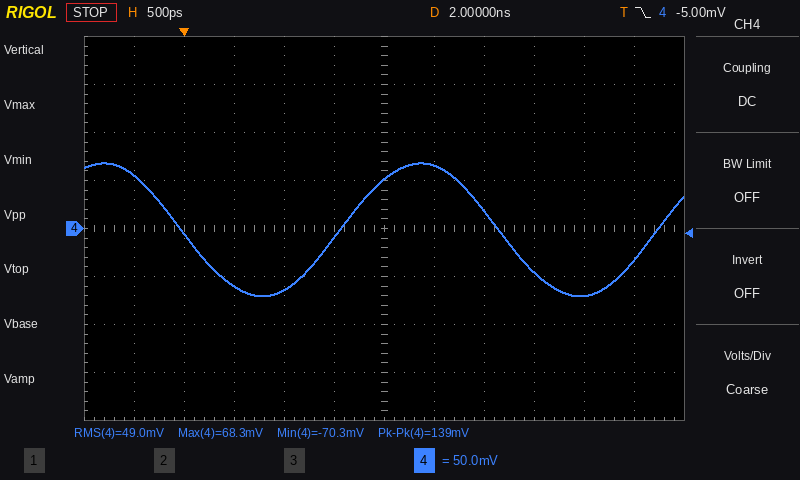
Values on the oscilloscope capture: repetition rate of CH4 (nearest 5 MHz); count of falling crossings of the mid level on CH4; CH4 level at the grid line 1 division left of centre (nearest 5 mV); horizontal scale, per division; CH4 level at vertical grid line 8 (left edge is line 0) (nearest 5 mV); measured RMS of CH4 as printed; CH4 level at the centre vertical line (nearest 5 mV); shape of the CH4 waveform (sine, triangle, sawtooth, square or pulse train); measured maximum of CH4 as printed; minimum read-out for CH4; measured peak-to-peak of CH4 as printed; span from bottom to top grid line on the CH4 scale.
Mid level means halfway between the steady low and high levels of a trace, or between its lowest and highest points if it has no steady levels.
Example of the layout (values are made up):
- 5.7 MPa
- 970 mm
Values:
- 315 MHz
- 2
- -10 mV
- 500 ps
- 20 mV
- 49.0 mV
- 50 mV
- sine
- 68.3 mV
- -70.3 mV
- 139 mV
- 400 mV
